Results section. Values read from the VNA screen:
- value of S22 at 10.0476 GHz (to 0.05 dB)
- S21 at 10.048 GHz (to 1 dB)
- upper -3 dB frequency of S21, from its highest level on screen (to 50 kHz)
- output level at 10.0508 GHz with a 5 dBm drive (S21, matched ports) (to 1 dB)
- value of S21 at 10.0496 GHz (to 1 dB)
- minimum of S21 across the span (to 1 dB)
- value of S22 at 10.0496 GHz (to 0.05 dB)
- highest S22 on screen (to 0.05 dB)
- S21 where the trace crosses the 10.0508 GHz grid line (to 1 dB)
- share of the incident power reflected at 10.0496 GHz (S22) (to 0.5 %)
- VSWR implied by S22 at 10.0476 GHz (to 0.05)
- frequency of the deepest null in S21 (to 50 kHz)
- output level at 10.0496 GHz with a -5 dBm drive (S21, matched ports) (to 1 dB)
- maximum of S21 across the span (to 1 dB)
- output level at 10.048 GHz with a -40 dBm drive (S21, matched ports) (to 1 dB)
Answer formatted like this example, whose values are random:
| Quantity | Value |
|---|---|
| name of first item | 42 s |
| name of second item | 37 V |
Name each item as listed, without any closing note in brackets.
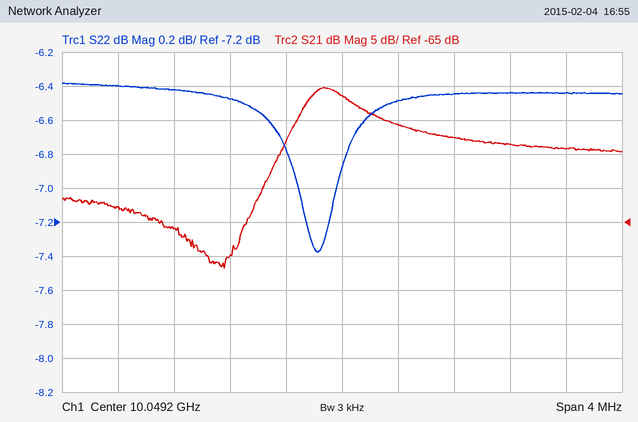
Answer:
| Quantity | Value |
|---|---|
| value of S22 at 10.0476 GHz | -6.40 dB |
| S21 at 10.048 GHz | -66 dB |
| upper -3 dB frequency of S21, from its highest level on screen | 10.04935 GHz |
| output level at 10.0508 GHz with a 5 dBm drive (S21, matched ports) | -49 dBm |
| value of S21 at 10.0496 GHz | -51 dB |
| minimum of S21 across the span | -72 dB |
| value of S22 at 10.0496 GHz | -6.50 dB |
| highest S22 on screen | -6.40 dB |
| S21 where the trace crosses the 10.0508 GHz grid line | -54 dB |
| share of the incident power reflected at 10.0496 GHz (S22) | 22.5 % |
| VSWR implied by S22 at 10.0476 GHz | 2.85 |
| frequency of the deepest null in S21 | 10.04835 GHz |
| output level at 10.0496 GHz with a -5 dBm drive (S21, matched ports) | -56 dBm |
| maximum of S21 across the span | -45 dB |
| output level at 10.048 GHz with a -40 dBm drive (S21, matched ports) | -106 dBm |
